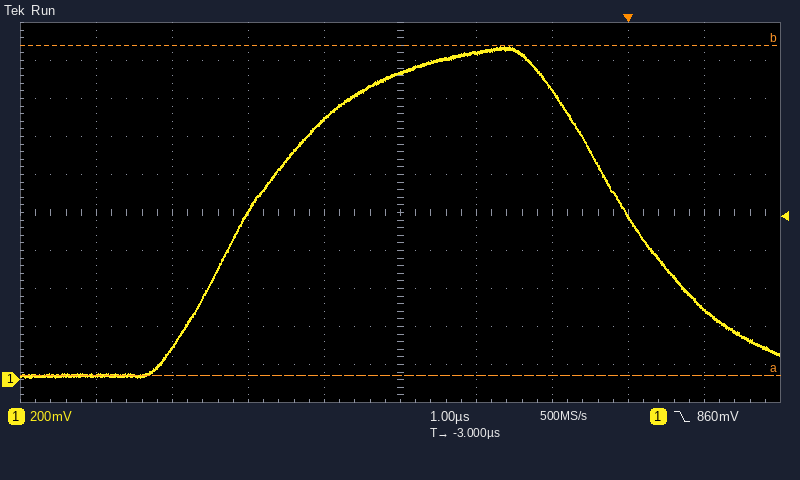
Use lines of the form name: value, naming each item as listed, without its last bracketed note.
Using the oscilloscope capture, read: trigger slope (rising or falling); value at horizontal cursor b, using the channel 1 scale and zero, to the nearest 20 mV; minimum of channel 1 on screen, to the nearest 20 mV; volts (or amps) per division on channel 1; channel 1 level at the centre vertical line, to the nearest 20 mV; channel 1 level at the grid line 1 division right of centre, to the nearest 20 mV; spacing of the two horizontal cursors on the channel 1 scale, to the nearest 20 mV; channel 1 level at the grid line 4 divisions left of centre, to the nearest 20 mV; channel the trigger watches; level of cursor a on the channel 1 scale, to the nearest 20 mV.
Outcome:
trigger slope: falling
value at horizontal cursor b, using the channel 1 scale and zero, to the nearest 20 mV: 1.76 V
minimum of channel 1 on screen, to the nearest 20 mV: 20 mV
volts (or amps) per division on channel 1: 200 mV
channel 1 level at the centre vertical line, to the nearest 20 mV: 1.62 V
channel 1 level at the grid line 1 division right of centre, to the nearest 20 mV: 1.72 V
spacing of the two horizontal cursors on the channel 1 scale, to the nearest 20 mV: 1.74 V
channel 1 level at the grid line 4 divisions left of centre, to the nearest 20 mV: 20 mV
channel the trigger watches: channel 1
level of cursor a on the channel 1 scale, to the nearest 20 mV: 20 mV
